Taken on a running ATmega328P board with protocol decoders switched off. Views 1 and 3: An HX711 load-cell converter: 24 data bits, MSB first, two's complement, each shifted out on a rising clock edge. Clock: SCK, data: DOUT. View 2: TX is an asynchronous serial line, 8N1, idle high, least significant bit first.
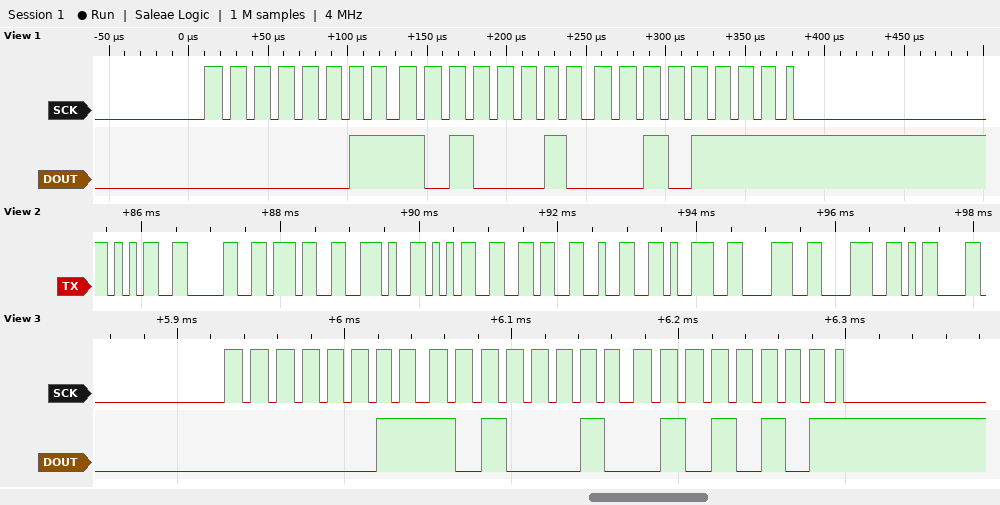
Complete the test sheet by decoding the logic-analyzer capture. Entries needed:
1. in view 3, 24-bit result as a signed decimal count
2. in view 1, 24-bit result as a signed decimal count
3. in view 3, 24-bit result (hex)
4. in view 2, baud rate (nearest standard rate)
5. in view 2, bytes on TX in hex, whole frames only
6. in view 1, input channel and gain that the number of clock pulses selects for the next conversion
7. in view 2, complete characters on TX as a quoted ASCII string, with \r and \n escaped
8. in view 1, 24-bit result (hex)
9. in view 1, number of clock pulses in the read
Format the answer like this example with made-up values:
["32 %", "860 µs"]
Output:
["238165", "238127", "0x03A255", "9600 baud", "35 30 37 2E 35 36 32 39 38 38 0D", "channel A, gain 128", "\"507.562988\\r\"", "0x03A22F", "25"]
